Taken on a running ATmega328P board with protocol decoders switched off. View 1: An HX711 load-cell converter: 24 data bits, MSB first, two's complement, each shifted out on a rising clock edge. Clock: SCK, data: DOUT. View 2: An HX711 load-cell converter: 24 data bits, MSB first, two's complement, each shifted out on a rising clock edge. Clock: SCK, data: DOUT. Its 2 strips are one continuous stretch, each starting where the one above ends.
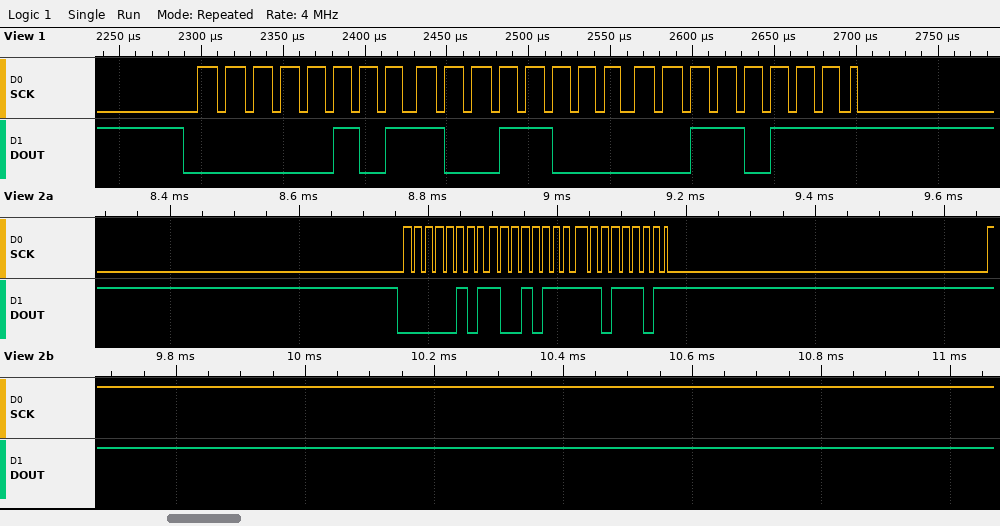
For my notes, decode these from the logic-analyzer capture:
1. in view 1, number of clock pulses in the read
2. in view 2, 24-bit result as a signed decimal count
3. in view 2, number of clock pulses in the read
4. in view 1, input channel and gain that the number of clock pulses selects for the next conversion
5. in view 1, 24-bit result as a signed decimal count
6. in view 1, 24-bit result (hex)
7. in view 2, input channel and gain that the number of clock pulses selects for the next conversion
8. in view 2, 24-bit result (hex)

25
366557
26
channel A, gain 128
366647
0x059837
channel B, gain 32
0x0597DD
